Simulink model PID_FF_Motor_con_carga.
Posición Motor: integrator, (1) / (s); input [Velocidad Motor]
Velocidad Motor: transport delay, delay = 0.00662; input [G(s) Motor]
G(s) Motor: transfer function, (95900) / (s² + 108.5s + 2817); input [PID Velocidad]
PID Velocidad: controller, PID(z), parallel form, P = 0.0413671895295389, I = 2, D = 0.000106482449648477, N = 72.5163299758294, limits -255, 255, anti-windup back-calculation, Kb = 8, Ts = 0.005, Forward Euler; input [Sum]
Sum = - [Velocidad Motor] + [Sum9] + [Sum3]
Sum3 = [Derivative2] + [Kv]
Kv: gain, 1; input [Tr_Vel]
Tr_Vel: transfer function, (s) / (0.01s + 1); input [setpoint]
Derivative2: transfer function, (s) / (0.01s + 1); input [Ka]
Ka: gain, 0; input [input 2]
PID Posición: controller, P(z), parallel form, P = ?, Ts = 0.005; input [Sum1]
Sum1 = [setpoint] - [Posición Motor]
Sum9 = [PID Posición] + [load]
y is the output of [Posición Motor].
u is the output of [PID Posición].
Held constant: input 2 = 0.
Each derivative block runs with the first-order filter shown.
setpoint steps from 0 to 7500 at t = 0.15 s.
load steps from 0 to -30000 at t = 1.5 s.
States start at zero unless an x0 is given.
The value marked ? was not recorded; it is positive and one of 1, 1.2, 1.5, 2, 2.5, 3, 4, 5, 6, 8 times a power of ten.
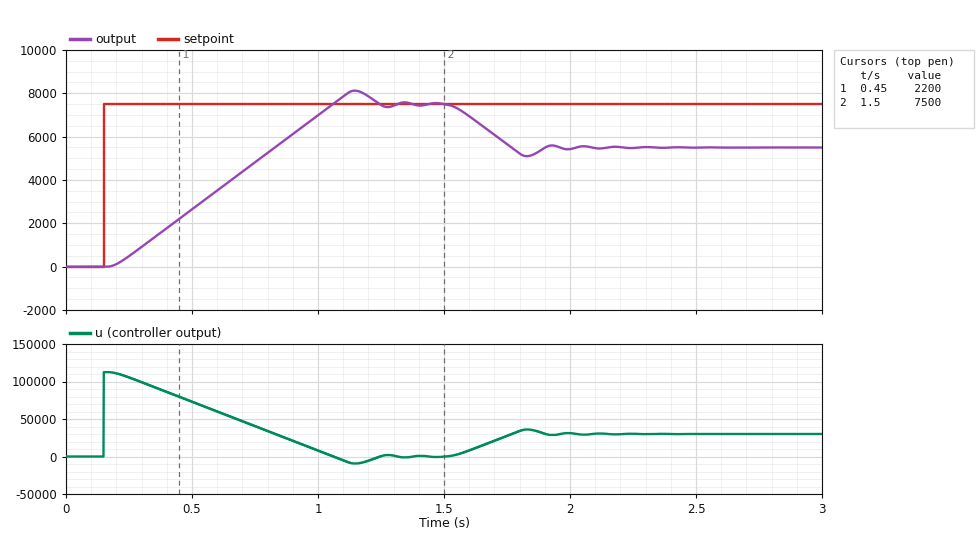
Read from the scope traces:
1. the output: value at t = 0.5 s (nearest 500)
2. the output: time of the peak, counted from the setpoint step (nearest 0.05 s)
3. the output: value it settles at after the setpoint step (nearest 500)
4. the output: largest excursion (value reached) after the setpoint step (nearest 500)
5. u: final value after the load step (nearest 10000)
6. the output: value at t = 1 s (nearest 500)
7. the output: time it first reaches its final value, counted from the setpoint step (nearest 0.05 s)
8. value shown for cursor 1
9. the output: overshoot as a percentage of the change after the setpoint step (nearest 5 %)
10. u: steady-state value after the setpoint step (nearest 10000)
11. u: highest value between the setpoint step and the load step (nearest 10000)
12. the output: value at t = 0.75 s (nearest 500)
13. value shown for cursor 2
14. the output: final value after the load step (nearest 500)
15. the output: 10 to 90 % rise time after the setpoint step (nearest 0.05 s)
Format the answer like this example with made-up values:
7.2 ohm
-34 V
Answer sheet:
2500
1.00 s
7500
8000
30000
7000
0.90 s
2200
10 %
0
110000
5000
7500
5500
0.70 s
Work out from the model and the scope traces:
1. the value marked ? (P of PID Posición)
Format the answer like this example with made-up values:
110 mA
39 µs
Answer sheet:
15
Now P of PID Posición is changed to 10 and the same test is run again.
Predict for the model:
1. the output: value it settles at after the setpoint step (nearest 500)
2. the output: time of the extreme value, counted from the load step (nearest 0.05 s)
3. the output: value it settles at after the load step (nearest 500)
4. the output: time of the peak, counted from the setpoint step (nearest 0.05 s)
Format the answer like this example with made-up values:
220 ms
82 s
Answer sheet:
7500
0.45 s
4500
0.95 s
